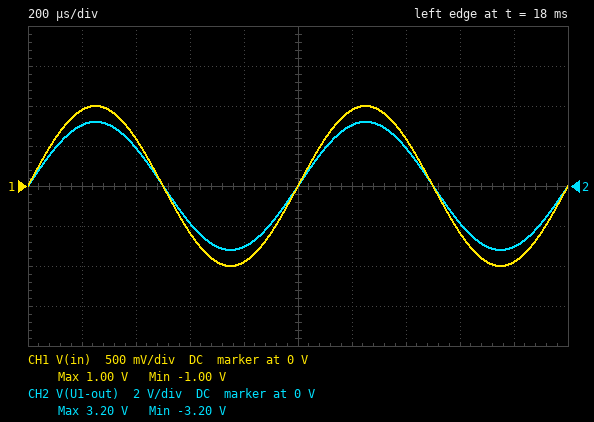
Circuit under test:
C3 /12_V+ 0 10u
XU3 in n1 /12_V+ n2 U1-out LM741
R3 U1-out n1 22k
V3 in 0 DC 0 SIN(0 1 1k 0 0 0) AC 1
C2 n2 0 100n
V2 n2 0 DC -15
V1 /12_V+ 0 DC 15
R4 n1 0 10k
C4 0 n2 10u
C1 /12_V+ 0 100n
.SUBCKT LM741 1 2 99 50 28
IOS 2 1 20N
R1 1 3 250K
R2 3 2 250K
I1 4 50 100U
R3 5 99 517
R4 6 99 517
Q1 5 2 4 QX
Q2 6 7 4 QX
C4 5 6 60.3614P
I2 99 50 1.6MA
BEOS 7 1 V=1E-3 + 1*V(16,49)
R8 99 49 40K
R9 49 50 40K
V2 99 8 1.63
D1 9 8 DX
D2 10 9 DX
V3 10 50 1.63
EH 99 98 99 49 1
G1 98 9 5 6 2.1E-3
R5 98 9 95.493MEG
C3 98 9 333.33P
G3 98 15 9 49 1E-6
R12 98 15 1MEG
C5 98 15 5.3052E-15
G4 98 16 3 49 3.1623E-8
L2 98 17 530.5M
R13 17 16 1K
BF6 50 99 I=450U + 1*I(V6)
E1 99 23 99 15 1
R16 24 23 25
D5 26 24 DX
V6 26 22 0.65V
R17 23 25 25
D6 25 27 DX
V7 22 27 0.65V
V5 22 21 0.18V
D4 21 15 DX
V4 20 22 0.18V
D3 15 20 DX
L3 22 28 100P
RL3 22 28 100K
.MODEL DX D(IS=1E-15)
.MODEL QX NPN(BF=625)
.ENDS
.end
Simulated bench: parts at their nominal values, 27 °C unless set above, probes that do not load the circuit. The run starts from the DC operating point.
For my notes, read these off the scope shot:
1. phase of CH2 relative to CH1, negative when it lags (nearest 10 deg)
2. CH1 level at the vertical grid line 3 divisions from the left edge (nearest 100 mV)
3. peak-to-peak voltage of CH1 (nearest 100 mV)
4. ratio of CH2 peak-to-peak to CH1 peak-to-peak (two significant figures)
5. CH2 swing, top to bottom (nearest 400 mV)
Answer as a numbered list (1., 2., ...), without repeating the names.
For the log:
1. 0 deg
2. -600 mV
3. 2.0 V
4. 3.2
5. 6.4 V
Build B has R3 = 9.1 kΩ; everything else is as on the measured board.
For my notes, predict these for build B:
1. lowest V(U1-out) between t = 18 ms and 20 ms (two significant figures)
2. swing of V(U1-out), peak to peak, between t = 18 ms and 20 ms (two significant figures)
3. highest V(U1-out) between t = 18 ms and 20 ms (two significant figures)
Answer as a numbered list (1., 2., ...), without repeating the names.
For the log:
1. -1.9 V
2. 3.8 V
3. 1.9 V
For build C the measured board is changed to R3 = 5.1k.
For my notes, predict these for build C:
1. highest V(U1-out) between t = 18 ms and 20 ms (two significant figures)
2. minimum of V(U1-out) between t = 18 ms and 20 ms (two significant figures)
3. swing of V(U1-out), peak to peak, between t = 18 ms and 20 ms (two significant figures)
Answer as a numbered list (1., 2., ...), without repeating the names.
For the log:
1. 1.5 V
2. -1.5 V
3. 3.0 V
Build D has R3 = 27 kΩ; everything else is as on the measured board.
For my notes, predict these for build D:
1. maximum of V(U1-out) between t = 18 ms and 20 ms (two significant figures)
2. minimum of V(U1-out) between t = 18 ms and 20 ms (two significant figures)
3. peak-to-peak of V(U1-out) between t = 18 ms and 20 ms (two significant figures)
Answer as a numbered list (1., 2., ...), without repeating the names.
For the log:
1. 3.7 V
2. -3.7 V
3. 7.4 V
